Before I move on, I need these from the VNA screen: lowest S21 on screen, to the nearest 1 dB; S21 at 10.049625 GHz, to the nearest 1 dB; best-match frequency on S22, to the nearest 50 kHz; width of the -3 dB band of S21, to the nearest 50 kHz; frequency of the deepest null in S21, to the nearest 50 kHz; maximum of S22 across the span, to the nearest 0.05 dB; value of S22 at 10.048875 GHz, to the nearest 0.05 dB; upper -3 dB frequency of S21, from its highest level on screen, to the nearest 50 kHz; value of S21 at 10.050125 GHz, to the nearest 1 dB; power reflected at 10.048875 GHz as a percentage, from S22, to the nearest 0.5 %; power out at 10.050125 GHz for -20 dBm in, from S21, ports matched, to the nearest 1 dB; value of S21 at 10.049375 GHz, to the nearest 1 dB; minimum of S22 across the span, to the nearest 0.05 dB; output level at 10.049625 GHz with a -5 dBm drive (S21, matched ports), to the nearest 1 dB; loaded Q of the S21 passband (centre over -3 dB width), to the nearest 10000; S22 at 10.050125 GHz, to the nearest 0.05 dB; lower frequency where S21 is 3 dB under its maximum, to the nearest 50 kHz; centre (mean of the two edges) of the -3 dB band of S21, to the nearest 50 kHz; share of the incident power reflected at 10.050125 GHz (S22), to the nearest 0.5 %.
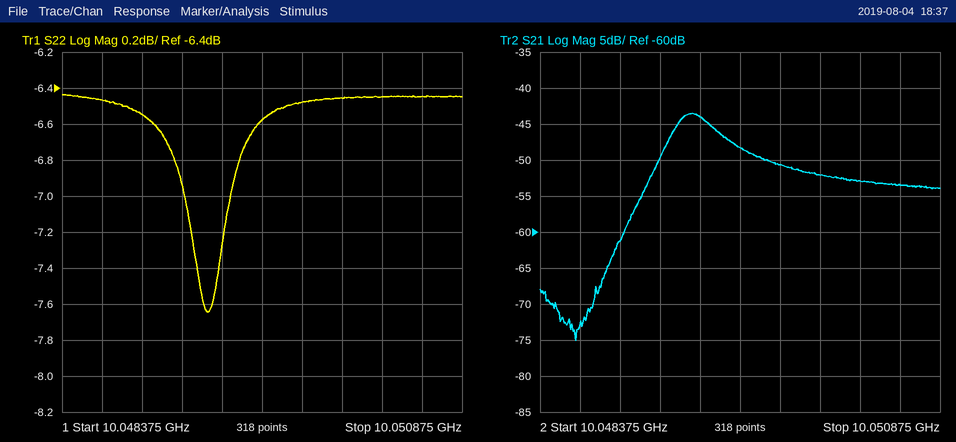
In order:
-75 dB
-48 dB
10.04930 GHz
300 kHz
10.04860 GHz
-6.45 dB
-6.55 dB
10.04950 GHz
-52 dB
22.0 %
-72 dBm
-44 dB
-7.65 dB
-53 dBm
30000
-6.45 dB
10.04920 GHz
10.04935 GHz
22.5 %
